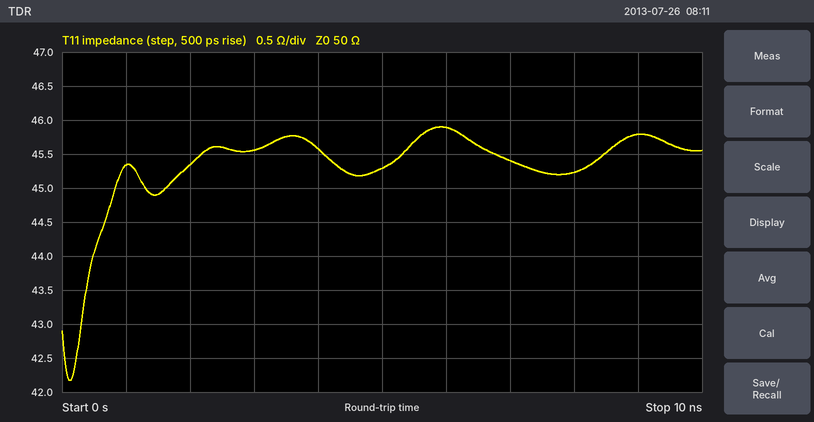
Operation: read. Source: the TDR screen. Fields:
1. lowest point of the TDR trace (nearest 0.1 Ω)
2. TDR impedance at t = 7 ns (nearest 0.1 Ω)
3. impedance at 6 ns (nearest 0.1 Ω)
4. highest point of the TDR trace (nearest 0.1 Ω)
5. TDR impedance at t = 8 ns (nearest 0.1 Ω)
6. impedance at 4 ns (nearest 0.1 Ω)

42.2 Ω
45.4 Ω
45.9 Ω
45.9 Ω
45.2 Ω
45.6 Ω
